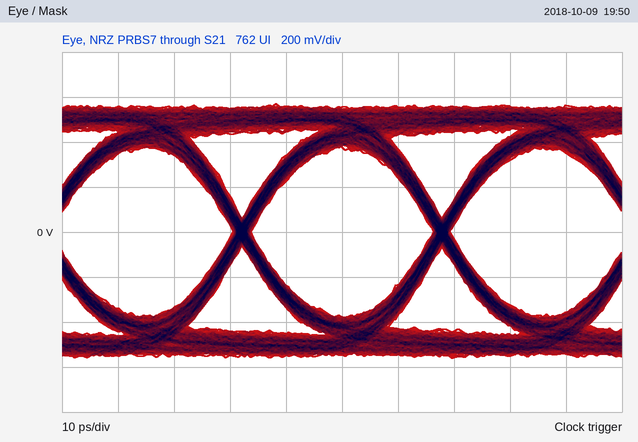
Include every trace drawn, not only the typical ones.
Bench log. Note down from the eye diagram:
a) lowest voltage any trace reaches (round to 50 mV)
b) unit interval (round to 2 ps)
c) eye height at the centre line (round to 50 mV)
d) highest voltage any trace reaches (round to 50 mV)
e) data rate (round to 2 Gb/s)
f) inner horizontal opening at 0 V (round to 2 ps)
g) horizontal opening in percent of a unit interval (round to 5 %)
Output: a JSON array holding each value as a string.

["-550 mV", "36 ps", "750 mV", "550 mV", "28 Gb/s", "32 ps", "90 %"]
